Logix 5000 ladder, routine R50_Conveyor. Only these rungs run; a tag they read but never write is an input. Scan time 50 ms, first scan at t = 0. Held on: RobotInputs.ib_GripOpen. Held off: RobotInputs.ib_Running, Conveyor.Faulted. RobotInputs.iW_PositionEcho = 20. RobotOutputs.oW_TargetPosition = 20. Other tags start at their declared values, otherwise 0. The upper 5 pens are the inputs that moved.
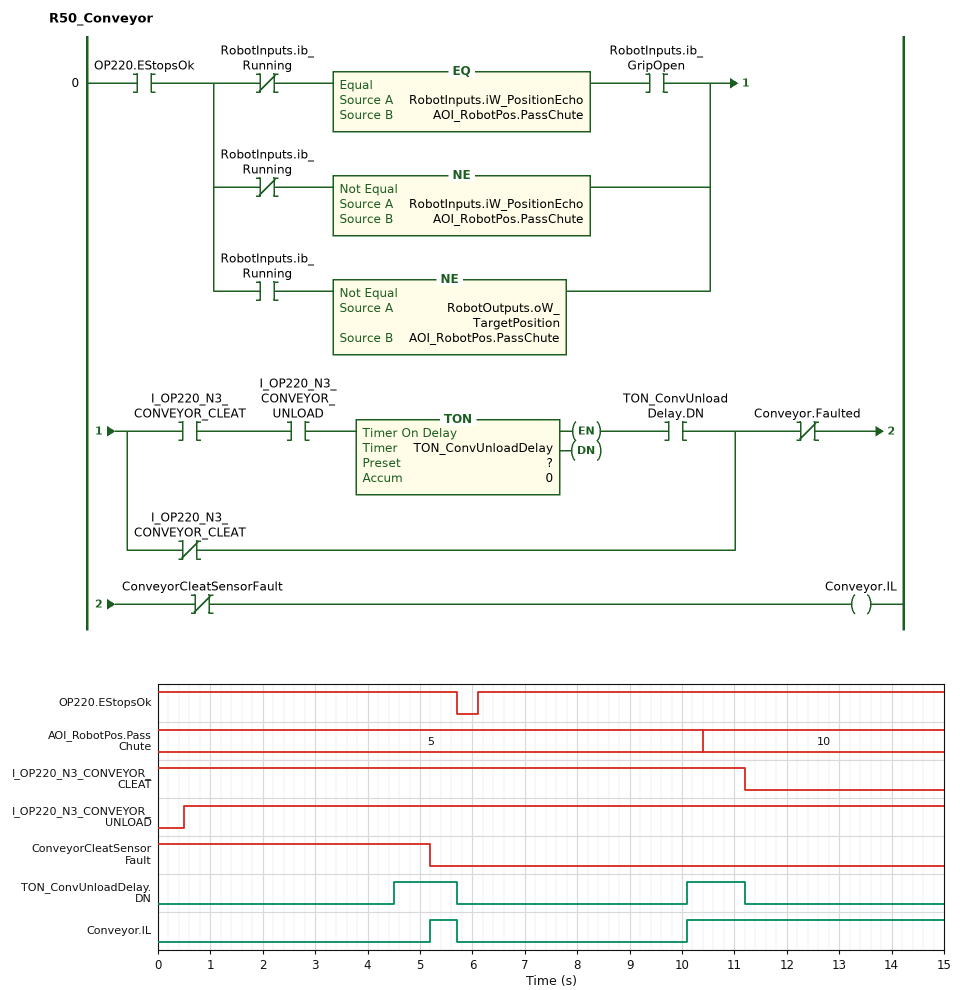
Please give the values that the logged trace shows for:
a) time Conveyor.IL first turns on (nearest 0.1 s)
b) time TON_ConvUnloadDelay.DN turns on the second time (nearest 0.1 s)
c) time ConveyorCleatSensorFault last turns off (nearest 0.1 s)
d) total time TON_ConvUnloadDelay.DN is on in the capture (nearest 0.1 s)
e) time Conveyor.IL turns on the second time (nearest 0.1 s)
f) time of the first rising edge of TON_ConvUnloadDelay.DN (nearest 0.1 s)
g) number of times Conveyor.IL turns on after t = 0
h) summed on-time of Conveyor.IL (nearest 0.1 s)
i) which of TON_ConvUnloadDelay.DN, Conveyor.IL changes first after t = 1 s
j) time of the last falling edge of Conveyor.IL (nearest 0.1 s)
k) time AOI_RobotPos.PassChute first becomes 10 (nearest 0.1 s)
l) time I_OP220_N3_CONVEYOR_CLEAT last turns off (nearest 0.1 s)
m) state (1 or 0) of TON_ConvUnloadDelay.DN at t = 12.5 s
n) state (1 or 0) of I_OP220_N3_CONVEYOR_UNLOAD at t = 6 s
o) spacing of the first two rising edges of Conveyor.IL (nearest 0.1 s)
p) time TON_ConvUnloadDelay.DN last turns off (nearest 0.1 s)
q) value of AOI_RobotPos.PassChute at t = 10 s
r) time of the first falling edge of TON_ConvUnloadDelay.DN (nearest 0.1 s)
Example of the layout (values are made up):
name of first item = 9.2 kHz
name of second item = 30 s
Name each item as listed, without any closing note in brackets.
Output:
time Conveyor.IL first turns on = 5.2 s
time TON_ConvUnloadDelay.DN turns on the second time = 10.1 s
time ConveyorCleatSensorFault last turns off = 5.2 s
total time TON_ConvUnloadDelay.DN is on in the capture = 2.3 s
time Conveyor.IL turns on the second time = 10.1 s
time of the first rising edge of TON_ConvUnloadDelay.DN = 4.5 s
number of times Conveyor.IL turns on after t = 0 = 2
summed on-time of Conveyor.IL = 5.4 s
which of TON_ConvUnloadDelay.DN, Conveyor.IL changes first after t = 1 s = TON_ConvUnloadDelay.DN
time of the last falling edge of Conveyor.IL = 5.7 s
time AOI_RobotPos.PassChute first becomes 10 = 10.4 s
time I_OP220_N3_CONVEYOR_CLEAT last turns off = 11.2 s
state (1 or 0) of TON_ConvUnloadDelay.DN at t = 12.5 s = 0
state (1 or 0) of I_OP220_N3_CONVEYOR_UNLOAD at t = 6 s = 1
spacing of the first two rising edges of Conveyor.IL = 4.9 s
time TON_ConvUnloadDelay.DN last turns off = 11.2 s
value of AOI_RobotPos.PassChute at t = 10 s = 5
time of the first falling edge of TON_ConvUnloadDelay.DN = 5.7 s
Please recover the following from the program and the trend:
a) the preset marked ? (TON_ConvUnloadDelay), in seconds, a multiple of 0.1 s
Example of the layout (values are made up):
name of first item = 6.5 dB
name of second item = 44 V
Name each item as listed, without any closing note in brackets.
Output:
the preset marked ? (TON_ConvUnloadDelay), in seconds, a multiple of 0.1 s = 4.0 s
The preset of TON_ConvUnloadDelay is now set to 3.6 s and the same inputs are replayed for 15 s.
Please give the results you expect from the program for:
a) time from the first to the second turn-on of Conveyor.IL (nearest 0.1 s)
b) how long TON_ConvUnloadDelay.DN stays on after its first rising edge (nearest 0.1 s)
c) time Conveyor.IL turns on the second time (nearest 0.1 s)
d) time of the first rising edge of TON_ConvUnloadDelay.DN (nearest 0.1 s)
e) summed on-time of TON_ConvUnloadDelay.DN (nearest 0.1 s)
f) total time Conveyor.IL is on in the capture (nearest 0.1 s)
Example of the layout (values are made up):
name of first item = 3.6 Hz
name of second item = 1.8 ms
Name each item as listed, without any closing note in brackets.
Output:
time from the first to the second turn-on of Conveyor.IL = 4.5 s
how long TON_ConvUnloadDelay.DN stays on after its first rising edge = 1.6 s
time Conveyor.IL turns on the second time = 9.7 s
time of the first rising edge of TON_ConvUnloadDelay.DN = 4.1 s
summed on-time of TON_ConvUnloadDelay.DN = 3.1 s
total time Conveyor.IL is on in the capture = 5.8 s
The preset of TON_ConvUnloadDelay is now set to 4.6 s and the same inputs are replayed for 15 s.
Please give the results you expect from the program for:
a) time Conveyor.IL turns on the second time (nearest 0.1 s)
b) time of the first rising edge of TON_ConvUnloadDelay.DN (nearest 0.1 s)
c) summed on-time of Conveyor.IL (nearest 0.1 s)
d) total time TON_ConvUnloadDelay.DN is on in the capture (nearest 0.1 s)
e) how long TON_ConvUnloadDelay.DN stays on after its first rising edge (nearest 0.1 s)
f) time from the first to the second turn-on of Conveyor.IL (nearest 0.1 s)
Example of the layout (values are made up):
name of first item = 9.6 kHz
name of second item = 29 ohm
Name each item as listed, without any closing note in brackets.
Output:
time Conveyor.IL turns on the second time = 10.7 s
time of the first rising edge of TON_ConvUnloadDelay.DN = 5.1 s
summed on-time of Conveyor.IL = 4.8 s
total time TON_ConvUnloadDelay.DN is on in the capture = 1.1 s
how long TON_ConvUnloadDelay.DN stays on after its first rising edge = 0.6 s
time from the first to the second turn-on of Conveyor.IL = 5.5 s
